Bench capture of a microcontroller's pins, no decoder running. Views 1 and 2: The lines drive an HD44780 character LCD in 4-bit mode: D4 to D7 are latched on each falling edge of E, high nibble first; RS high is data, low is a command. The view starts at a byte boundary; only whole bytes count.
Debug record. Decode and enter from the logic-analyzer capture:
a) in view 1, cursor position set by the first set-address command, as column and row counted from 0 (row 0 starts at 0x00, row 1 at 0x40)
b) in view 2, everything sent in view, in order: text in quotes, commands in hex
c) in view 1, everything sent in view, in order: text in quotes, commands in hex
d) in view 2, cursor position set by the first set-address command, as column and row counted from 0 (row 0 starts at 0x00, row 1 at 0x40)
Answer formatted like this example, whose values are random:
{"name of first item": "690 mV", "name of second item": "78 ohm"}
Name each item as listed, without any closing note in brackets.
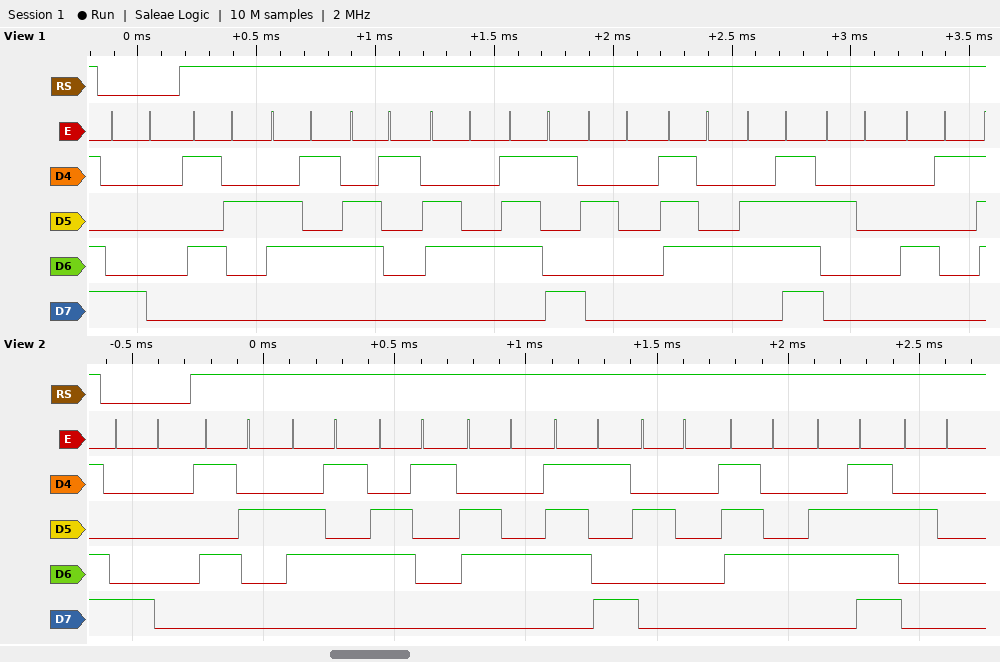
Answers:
{"in view 1, cursor position set by the first set-address command, as column and row counted from 0": "column 0, row 0", "in view 2, everything sent in view, in order: text in quotes, commands in hex": "0x80 \"Ready to \"", "in view 1, everything sent in view, in order: text in quotes, commands in hex": "0x80 \"Ready to A\"", "in view 2, cursor position set by the first set-address command, as column and row counted from 0": "column 0, row 0"}
